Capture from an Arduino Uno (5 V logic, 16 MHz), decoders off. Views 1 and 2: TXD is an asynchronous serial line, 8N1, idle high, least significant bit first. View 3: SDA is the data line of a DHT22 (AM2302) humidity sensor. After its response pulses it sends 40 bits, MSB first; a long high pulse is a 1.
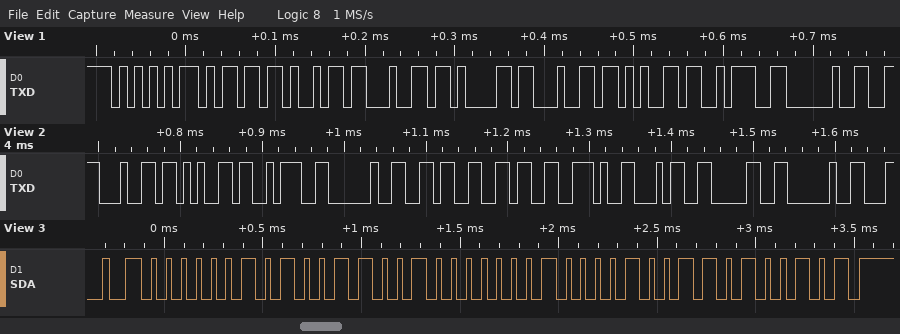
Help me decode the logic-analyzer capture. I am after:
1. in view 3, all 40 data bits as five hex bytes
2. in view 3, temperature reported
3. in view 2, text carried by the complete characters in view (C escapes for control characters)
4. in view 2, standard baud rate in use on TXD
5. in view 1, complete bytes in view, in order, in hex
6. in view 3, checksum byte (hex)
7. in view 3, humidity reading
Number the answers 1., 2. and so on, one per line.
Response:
1. 02 99 01 09 A5
2. 26.5 °C
3. "de: 66.40 "
4. 115200 baud
5. 55 6D 69 64 61 64 65 3A 20
6. 0xA5
7. 66.5 %
